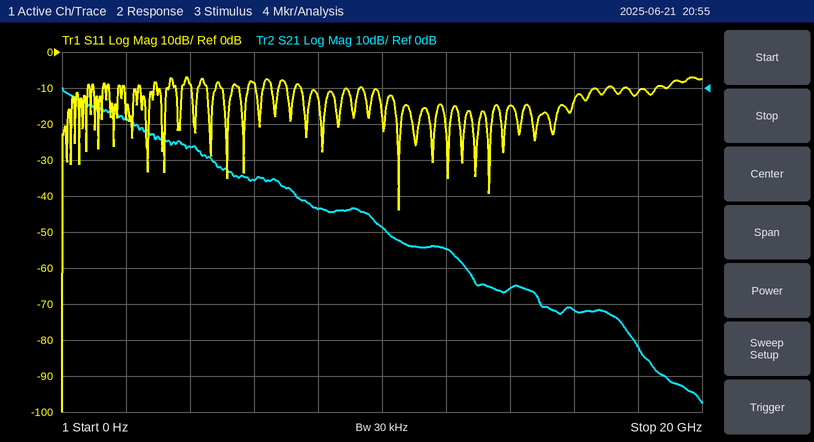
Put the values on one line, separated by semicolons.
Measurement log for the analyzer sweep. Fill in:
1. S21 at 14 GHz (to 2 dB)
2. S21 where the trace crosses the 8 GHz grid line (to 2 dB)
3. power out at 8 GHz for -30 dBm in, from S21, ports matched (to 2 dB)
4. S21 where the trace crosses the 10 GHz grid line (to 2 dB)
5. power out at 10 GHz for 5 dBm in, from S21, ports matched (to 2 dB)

-56 dB; -34 dB; -64 dBm; -38 dB; -34 dBm
